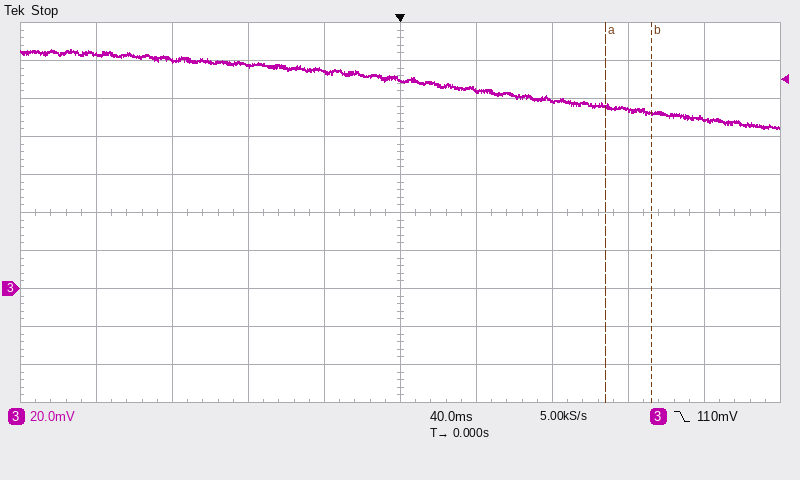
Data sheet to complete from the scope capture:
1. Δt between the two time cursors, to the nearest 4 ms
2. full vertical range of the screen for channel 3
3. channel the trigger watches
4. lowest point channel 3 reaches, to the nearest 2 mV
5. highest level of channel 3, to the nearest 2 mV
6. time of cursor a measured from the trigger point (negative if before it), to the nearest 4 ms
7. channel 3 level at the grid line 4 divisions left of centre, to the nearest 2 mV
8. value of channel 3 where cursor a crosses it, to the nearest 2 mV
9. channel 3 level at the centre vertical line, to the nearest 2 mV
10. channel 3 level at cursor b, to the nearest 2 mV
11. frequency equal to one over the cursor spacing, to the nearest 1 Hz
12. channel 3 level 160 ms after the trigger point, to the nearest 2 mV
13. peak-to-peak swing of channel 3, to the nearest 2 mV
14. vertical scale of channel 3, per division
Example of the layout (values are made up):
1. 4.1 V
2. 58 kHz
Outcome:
1. 24 ms
2. 200 mV
3. channel 3
4. 84 mV
5. 126 mV
6. +108 ms
7. 124 mV
8. 96 mV
9. 110 mV
10. 92 mV
11. 42 Hz
12. 90 mV
13. 42 mV
14. 20 mV
